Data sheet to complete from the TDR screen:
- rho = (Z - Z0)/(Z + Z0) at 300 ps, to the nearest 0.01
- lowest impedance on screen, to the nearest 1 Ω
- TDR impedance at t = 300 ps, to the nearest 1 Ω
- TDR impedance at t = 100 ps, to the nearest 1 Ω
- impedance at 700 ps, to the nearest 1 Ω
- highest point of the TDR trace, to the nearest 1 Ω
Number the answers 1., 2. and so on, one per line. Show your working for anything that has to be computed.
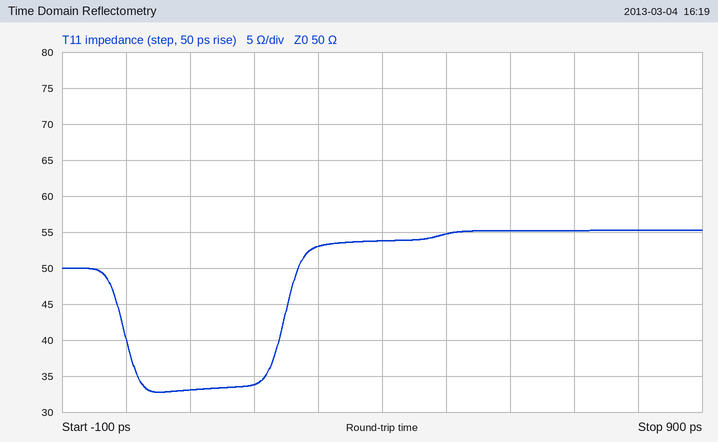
1. (53 − 50)/(53 + 50) ≈ +0.03
2. 33 Ω
3. 53 Ω
4. 33 Ω
5. 55 Ω
6. 55 Ω
